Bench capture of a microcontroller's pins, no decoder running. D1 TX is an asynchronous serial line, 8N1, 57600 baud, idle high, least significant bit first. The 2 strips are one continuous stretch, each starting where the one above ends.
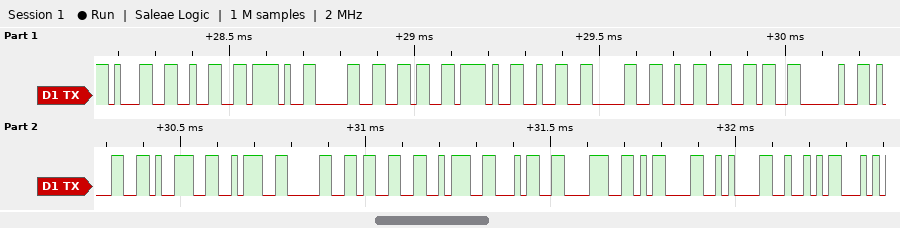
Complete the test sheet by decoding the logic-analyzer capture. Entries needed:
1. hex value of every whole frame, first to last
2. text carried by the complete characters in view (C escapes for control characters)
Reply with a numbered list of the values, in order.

1. 0x31 0x32 0x2F 0x30 0x36 0x2F 0x32 0x30 0x32 0x36 0x20 0x31 0x39 0x3A 0x30 0x33 0x3A 0x34 0x38 0x0D 0x0A 0x52
2. "12/06/2026 19:03:48\r\nR"
